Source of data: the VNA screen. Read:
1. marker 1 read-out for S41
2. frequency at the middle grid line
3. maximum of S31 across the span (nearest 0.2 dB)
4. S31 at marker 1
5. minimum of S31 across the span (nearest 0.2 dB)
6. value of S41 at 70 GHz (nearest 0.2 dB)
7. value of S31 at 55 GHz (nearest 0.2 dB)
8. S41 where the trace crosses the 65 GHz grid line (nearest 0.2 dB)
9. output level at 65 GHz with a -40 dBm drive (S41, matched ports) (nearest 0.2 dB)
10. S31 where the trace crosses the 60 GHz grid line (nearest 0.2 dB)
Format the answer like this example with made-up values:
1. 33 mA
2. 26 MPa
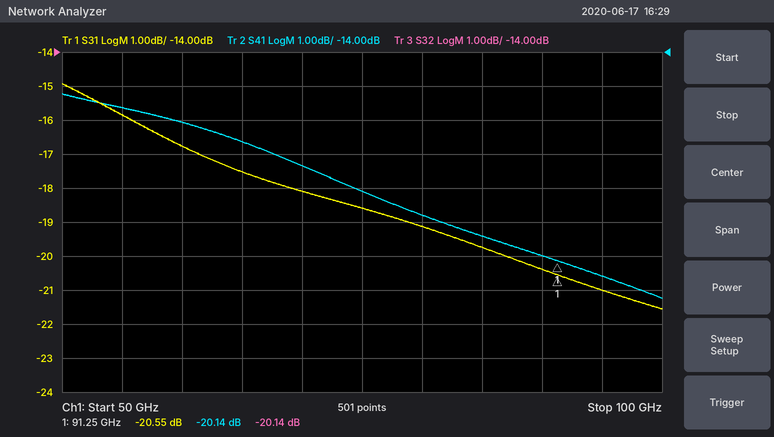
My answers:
1. -20.14 dB
2. 75 GHz
3. -15.0 dB
4. -20.55 dB
5. -21.6 dB
6. -17.4 dB
7. -15.8 dB
8. -16.6 dB
9. -56.6 dBm
10. -16.8 dB
